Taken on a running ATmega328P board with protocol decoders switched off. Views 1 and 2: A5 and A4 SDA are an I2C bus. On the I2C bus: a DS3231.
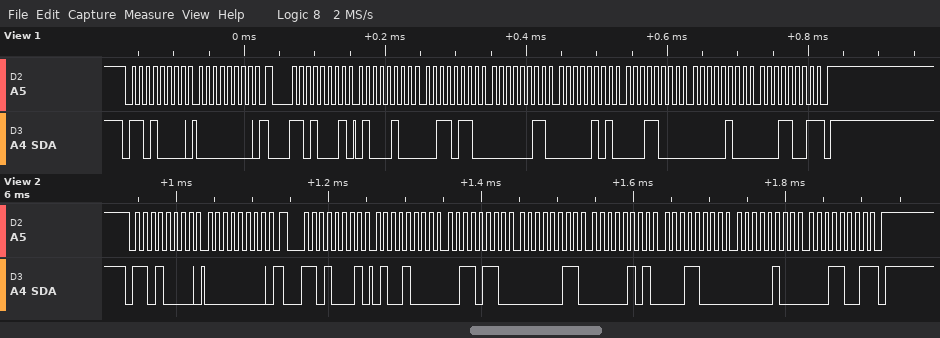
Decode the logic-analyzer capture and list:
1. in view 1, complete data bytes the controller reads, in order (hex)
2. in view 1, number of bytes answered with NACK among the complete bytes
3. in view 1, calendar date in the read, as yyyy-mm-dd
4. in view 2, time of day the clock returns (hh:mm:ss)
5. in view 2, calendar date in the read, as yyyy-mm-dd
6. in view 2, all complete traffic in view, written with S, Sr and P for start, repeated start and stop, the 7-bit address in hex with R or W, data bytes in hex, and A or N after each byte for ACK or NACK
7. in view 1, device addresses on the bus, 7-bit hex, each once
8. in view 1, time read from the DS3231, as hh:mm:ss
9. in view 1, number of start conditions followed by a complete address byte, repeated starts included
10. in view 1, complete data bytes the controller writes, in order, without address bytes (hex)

44 36 03 05 18 04 19
1
2019-04-18
03:36:48
2019-04-18
S 68W A 00 A Sr 68R A 48 A 36 A 03 A 05 A 18 A 04 A 19 N P
0x68
03:36:44
2
00
